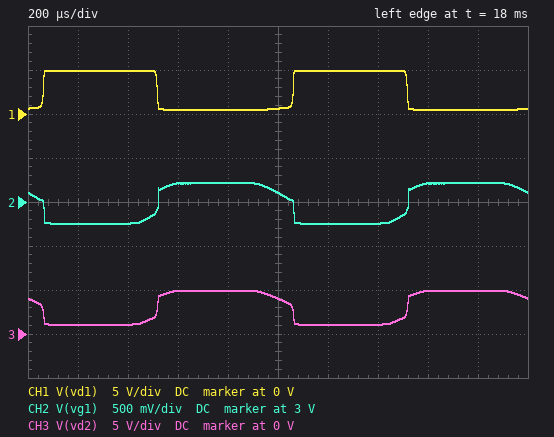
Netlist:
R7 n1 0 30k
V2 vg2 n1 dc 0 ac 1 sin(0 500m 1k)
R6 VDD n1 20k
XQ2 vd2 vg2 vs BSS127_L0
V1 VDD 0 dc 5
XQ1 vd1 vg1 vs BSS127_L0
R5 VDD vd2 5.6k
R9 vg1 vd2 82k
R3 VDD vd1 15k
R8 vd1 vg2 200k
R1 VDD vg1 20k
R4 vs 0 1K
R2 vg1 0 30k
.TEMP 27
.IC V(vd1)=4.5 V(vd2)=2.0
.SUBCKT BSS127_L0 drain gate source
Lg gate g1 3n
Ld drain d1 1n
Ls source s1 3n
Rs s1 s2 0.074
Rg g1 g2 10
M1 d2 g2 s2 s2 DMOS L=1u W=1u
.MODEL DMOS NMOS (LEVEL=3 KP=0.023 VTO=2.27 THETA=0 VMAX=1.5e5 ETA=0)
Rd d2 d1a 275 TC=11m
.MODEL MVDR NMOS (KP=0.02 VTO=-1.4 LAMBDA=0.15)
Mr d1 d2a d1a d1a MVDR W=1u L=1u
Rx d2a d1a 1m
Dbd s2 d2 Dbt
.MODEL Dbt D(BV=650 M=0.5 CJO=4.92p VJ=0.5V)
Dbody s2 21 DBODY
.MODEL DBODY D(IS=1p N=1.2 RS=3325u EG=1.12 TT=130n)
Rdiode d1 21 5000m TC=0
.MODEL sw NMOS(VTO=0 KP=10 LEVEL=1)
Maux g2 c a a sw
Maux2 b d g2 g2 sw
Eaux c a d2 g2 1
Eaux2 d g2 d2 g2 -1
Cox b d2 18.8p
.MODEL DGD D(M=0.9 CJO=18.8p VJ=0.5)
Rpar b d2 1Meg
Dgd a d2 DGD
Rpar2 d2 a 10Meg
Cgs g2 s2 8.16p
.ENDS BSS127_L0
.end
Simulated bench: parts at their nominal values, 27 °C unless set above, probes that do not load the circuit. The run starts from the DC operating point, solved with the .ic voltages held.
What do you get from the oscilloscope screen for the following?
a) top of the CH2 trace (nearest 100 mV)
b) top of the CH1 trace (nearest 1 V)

3.2 V
5 V
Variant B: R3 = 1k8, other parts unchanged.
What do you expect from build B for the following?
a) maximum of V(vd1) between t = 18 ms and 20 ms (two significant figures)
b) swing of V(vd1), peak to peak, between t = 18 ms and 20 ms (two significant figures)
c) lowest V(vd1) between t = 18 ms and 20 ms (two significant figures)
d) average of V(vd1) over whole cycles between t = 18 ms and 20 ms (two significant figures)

5.0 V
1.3 V
3.7 V
4.4 V
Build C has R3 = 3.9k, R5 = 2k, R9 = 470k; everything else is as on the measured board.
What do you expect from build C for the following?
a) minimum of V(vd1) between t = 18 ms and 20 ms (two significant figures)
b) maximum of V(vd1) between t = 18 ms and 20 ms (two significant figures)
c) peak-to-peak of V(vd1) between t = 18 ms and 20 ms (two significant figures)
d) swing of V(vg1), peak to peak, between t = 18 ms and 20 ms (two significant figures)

2.9 V
5.0 V
2.1 V
46 mV
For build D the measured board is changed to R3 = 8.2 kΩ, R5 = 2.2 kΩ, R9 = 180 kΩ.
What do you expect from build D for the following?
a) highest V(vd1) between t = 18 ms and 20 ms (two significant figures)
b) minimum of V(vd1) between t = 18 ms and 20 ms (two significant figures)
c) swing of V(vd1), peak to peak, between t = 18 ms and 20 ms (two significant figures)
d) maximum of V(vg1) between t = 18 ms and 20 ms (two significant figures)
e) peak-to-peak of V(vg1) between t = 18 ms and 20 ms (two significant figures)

4.9 V
780 mV
4.2 V
3.1 V
100 mV
